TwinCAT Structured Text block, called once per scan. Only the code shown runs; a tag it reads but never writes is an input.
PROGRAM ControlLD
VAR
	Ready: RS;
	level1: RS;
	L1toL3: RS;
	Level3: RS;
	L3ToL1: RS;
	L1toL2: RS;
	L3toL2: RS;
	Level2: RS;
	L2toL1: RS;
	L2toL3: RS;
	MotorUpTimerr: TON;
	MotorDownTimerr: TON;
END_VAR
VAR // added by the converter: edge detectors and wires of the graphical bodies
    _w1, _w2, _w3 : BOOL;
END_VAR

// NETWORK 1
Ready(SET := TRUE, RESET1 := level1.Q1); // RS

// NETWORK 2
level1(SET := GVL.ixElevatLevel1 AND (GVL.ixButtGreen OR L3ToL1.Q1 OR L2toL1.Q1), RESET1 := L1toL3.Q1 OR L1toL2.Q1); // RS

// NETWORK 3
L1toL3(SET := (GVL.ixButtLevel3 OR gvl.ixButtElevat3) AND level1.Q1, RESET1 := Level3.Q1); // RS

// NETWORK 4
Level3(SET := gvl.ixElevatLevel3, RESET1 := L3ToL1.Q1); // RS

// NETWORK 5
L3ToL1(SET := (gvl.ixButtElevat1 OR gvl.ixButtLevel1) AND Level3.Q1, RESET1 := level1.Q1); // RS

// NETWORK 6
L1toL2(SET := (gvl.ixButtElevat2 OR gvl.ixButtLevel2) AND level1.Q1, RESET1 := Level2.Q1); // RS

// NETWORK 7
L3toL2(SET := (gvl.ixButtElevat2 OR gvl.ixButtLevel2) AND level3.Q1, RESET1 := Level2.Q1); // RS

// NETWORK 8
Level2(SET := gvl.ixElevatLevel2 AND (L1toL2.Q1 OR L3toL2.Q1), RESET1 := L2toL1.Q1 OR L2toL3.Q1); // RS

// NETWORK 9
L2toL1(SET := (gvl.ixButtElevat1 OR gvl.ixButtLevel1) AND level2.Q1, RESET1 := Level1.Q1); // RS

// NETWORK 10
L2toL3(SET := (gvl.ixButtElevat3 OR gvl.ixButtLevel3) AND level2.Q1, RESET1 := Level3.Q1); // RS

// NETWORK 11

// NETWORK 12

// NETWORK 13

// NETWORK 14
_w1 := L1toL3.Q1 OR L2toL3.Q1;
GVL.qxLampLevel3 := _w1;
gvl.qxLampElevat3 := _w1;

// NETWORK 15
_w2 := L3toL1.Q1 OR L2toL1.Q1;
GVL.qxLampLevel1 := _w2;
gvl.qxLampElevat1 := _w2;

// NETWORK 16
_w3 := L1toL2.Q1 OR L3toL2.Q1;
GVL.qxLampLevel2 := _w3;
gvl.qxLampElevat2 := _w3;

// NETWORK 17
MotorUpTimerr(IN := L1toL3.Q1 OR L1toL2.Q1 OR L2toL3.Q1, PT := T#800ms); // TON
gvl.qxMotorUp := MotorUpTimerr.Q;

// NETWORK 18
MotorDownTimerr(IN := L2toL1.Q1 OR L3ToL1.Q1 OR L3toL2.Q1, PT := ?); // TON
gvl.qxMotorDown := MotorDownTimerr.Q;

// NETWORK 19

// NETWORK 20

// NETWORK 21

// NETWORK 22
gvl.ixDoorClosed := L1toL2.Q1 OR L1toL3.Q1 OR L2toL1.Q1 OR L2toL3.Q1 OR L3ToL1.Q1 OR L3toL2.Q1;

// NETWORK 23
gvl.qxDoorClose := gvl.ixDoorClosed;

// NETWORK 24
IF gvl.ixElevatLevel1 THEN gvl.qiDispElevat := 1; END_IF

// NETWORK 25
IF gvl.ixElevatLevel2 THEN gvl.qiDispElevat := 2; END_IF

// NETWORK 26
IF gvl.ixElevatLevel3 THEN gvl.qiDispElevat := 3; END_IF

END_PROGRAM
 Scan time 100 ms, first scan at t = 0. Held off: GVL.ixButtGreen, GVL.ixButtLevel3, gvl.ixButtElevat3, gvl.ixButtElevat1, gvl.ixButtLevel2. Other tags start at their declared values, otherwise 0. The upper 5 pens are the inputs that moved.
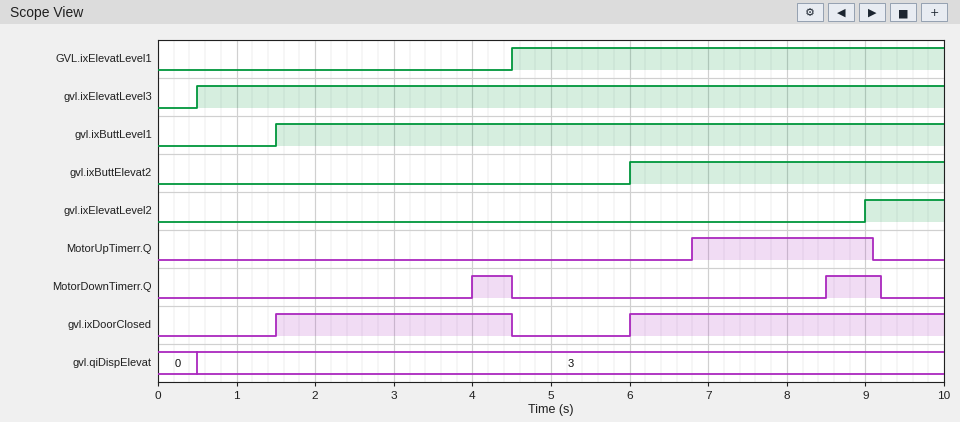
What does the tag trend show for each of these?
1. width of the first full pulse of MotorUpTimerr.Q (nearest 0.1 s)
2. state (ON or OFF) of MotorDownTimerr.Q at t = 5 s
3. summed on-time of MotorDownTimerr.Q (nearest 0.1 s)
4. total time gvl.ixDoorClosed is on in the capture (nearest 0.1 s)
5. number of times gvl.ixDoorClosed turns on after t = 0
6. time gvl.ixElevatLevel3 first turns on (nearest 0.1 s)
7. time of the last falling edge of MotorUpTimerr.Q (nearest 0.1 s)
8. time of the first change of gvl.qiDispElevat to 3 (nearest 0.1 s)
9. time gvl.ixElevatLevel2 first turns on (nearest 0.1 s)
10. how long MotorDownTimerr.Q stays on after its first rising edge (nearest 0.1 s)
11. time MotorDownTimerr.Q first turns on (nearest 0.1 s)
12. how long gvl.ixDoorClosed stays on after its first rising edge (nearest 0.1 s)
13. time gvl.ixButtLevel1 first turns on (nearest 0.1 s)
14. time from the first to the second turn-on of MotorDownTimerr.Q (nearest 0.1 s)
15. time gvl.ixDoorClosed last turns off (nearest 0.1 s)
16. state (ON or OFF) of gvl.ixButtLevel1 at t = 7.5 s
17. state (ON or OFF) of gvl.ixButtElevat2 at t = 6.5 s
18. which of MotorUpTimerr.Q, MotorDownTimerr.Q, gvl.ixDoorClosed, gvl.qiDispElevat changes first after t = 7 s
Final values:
2.3 s
OFF
1.2 s
7.0 s
2
0.5 s
9.1 s
0.5 s
9.0 s
0.5 s
4.0 s
3.0 s
1.5 s
4.5 s
4.5 s
ON
ON
MotorDownTimerr.Q
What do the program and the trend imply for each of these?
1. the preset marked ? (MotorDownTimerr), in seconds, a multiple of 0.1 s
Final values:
2.5 s
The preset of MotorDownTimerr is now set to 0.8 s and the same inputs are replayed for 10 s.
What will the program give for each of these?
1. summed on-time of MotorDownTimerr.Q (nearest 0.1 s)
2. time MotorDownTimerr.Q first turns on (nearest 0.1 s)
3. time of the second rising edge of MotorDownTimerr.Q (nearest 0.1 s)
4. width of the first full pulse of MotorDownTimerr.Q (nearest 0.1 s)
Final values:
4.6 s
2.3 s
6.8 s
2.2 s
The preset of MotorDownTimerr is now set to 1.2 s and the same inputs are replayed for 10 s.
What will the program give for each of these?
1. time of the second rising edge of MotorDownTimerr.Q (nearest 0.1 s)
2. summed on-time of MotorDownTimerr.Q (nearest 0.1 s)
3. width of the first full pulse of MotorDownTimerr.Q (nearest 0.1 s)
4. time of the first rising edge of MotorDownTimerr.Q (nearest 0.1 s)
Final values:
7.2 s
3.8 s
1.8 s
2.7 s
